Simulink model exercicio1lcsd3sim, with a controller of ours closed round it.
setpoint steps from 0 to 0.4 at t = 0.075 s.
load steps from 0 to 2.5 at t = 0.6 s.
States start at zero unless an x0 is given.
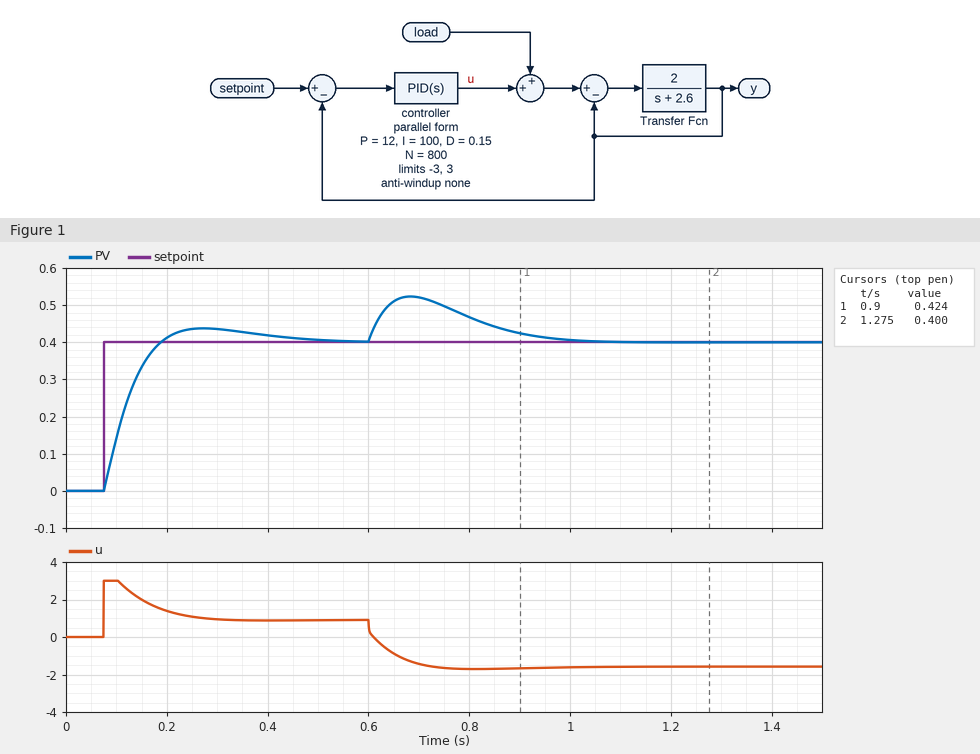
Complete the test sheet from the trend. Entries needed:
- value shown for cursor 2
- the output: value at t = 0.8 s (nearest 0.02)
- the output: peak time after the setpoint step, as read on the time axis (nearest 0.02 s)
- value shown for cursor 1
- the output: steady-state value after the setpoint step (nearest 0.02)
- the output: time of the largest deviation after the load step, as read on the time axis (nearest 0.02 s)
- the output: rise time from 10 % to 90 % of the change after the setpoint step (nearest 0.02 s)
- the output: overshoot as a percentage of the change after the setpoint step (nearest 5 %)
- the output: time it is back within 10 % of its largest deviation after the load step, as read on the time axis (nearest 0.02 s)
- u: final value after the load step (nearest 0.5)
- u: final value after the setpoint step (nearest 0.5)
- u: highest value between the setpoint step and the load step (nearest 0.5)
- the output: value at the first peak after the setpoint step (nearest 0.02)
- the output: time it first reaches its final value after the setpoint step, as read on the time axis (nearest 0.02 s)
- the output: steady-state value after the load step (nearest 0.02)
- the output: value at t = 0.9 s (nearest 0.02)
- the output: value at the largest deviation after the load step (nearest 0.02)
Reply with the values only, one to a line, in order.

0.400
0.46
0.28 s
0.424
0.40
0.68 s
0.08 s
10 %
0.96 s
-1.5
1.0
3.0
0.44
0.18 s
0.40
0.42
0.52
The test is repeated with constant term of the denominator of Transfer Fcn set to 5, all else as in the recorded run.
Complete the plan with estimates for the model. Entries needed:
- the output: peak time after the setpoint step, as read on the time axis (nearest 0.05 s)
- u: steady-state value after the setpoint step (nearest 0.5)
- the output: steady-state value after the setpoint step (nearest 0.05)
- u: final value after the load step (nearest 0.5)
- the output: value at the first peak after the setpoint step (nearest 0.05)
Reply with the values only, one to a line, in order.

0.30 s
1.5
0.40
-1.0
0.40
